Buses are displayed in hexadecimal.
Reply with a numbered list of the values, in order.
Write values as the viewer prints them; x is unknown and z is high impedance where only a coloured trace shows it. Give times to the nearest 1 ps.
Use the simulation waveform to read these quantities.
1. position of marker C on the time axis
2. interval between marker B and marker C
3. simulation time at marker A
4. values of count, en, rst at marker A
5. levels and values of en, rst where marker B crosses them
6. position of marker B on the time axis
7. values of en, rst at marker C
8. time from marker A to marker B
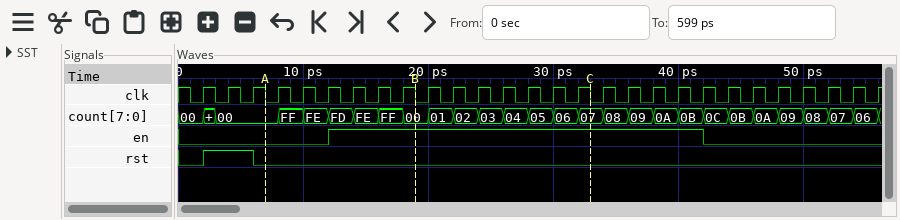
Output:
1. 33 ps
2. 14 ps
3. 7 ps
4. count=00, en=0, rst=0
5. en=1, rst=0
6. 19 ps
7. en=1, rst=0
8. 12 ps
